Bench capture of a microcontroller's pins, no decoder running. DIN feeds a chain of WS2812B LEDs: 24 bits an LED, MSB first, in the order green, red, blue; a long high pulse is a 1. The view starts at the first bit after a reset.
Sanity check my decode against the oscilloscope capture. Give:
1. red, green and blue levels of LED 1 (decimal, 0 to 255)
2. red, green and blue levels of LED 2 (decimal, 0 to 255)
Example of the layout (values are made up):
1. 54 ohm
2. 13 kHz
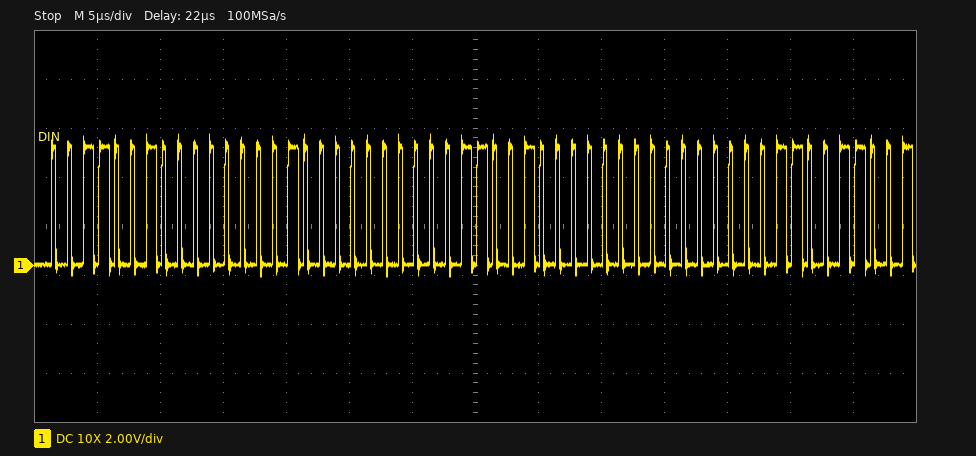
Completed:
1. 1, 50, 0
2. 0, 50, 3
